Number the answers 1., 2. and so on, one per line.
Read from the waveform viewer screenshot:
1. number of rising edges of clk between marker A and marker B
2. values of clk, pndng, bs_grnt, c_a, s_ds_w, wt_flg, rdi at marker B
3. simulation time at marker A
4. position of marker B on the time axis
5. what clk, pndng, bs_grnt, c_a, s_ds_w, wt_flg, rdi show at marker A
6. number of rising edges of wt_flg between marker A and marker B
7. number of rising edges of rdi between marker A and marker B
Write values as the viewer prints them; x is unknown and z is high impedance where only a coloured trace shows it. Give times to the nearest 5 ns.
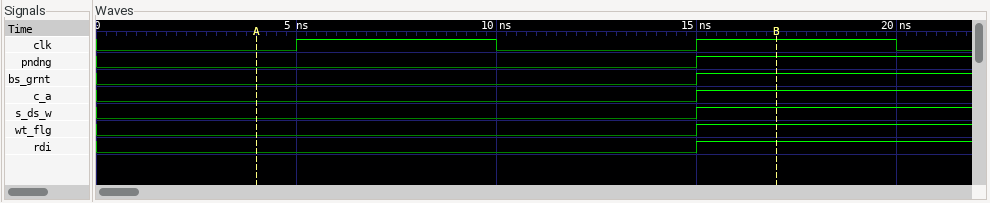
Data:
1. 2
2. clk=1, pndng=1, bs_grnt=1, c_a=1, s_ds_w=1, wt_flg=1, rdi=1
3. 5 ns
4. 15 ns
5. clk=0, pndng=0, bs_grnt=0, c_a=0, s_ds_w=0, wt_flg=0, rdi=0
6. 1
7. 1
